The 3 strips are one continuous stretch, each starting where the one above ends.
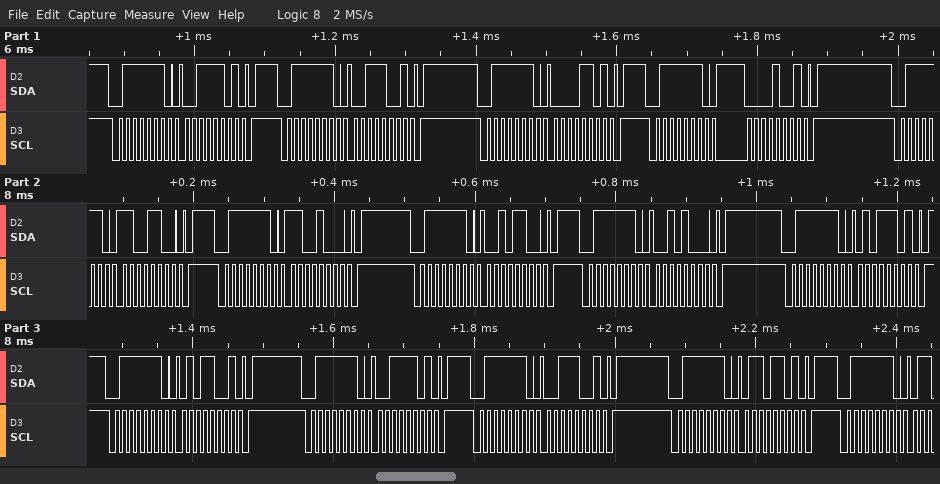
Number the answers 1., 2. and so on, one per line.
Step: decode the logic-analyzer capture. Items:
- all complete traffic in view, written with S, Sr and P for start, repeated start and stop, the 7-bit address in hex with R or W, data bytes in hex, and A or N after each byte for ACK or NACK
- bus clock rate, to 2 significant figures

1. S 3FW A 3D A P S 3FW A 39 A P S 3FW A 0D A P S 3FW A 09 A P S 3FW A CC A P S 3FW A C8 A P S 3FW A 2C A P S 3FW A 28 A P S 3FW A 5D A P S 3FW A 59 A P S 3FW A 3D A P S 3FW A 39 A P S 3FW A 6D A P S 3FW A
2. 100 kHz
